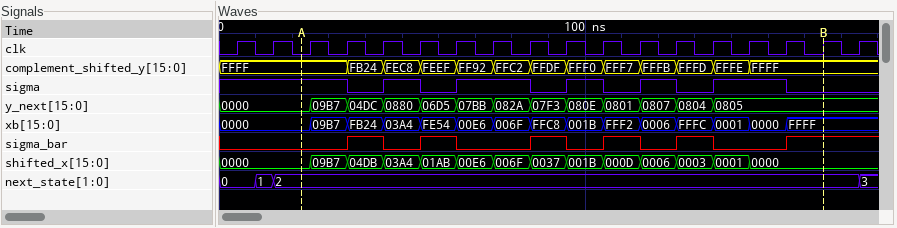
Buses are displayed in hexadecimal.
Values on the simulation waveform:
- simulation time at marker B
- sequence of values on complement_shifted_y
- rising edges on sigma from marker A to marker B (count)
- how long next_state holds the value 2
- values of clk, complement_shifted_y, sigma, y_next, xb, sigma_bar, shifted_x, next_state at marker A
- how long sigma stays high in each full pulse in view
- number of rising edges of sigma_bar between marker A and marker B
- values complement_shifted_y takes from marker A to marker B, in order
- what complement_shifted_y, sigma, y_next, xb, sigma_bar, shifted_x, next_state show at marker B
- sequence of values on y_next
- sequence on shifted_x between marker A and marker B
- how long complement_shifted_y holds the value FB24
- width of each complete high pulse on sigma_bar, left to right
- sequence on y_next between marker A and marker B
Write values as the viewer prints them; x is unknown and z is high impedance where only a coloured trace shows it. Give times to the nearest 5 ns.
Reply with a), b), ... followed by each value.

a) 165 ns
b) FFFF, FB24, FEC8, FEEF, FF92, FFC2, FFDF, FFF0, FFF7, FFFB, FFFD, FFFE, FFFF
c) 5
d) 160 ns
e) clk=0, complement_shifted_y=FFFF, sigma=1, y_next=0000, xb=0000, sigma_bar=0, shifted_x=0000, next_state=2
f) 10 ns, 20 ns, 10 ns, 10 ns, 20 ns
g) 6
h) FFFF, FB24, FEC8, FEEF, FF92, FFC2, FFDF, FFF0, FFF7, FFFB, FFFD, FFFE, FFFF
i) complement_shifted_y=FFFF, sigma=0, y_next=0805, xb=FFFF, sigma_bar=1, shifted_x=0000, next_state=2
j) 0000, 09B7, 04DC, 0880, 06D5, 07BB, 082A, 07F3, 080E, 0801, 0807, 0804, 0805
k) 0000, 09B7, 04DB, 03A4, 01AB, 00E6, 006F, 0037, 001B, 000D, 0006, 0003, 0001, 0000
l) 10 ns
m) 10 ns, 10 ns, 10 ns, 10 ns, 10 ns
n) 0000, 09B7, 04DC, 0880, 06D5, 07BB, 082A, 07F3, 080E, 0801, 0807, 0804, 0805
